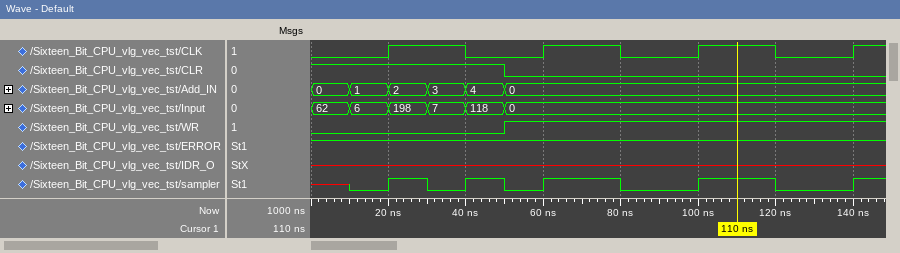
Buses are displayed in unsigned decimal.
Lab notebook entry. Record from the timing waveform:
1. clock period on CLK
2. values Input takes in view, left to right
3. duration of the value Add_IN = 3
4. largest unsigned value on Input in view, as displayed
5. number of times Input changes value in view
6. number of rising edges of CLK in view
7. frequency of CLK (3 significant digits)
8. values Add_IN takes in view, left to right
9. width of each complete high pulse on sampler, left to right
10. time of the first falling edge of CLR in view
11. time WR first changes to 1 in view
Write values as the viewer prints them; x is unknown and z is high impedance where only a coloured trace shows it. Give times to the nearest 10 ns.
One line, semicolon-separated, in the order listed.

40 ns; 62, 6, 198, 7, 118, 0; 10 ns; 198; 5; 4; 25.0 MHz; 0, 1, 2, 3, 4, 0; 10 ns, 10 ns, 20 ns, 20 ns; 50 ns; 50 ns
